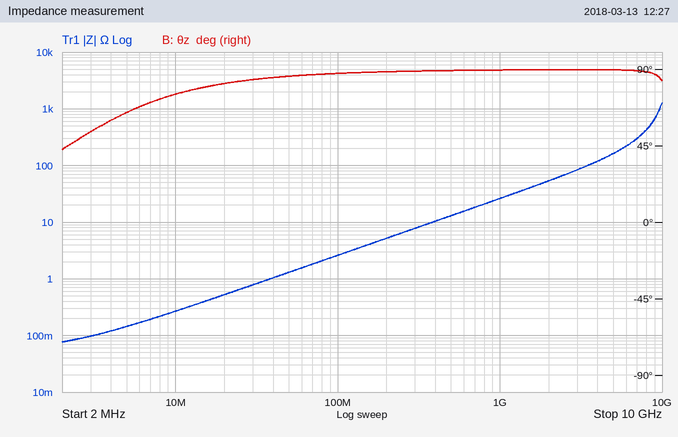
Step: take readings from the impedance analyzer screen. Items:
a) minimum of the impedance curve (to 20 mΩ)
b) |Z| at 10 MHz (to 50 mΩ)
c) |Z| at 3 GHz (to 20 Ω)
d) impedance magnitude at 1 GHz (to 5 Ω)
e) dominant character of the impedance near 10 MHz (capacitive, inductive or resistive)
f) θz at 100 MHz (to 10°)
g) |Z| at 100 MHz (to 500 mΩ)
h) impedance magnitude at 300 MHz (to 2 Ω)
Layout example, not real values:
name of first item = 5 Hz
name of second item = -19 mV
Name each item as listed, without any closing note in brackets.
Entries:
minimum of the impedance curve = 80 mΩ
|Z| at 10 MHz = 250 mΩ
|Z| at 3 GHz = 80 Ω
impedance magnitude at 1 GHz = 25 Ω
dominant character of the impedance near 10 MHz = inductive
θz at 100 MHz = 90°
|Z| at 100 MHz = 2.5 Ω
impedance magnitude at 300 MHz = 8 Ω
